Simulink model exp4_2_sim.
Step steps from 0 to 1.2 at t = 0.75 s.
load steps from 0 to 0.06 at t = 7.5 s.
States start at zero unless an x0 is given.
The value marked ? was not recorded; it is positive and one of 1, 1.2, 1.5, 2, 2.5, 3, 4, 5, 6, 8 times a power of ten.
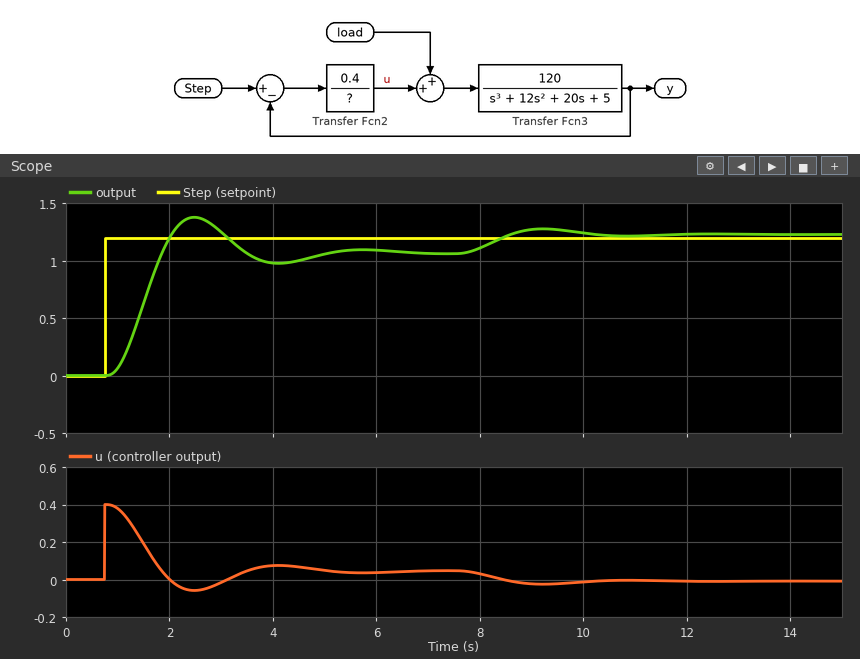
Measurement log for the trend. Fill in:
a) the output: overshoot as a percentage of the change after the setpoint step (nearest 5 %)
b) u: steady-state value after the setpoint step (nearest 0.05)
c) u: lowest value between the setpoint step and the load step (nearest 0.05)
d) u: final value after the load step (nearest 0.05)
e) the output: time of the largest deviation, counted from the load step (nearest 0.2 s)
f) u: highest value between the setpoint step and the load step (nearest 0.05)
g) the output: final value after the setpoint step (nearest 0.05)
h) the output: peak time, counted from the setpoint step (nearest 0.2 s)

30 %
0.05
-0.05
0.00
1.8 s
0.40
1.05
1.8 s
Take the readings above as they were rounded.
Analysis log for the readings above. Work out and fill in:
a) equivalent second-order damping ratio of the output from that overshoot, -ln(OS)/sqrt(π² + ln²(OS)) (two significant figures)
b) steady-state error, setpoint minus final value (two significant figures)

0.36
0.15
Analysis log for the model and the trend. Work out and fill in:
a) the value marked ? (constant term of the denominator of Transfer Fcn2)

1.2
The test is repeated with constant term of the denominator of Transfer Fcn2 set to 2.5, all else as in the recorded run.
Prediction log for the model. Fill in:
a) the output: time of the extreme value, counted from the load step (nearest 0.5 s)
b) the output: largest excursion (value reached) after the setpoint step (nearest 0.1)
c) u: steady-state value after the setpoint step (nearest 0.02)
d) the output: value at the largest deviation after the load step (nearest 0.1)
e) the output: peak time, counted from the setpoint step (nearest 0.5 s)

2.5 s
1.1
0.04
1.3
2.5 s
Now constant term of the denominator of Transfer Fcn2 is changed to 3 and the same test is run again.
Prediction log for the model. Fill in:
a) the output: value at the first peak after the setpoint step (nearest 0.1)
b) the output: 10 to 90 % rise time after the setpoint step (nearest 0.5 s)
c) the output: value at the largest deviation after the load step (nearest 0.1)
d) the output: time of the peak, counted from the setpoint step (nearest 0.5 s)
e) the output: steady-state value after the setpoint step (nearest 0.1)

1.0
1.5 s
1.3
3.0 s
0.9
